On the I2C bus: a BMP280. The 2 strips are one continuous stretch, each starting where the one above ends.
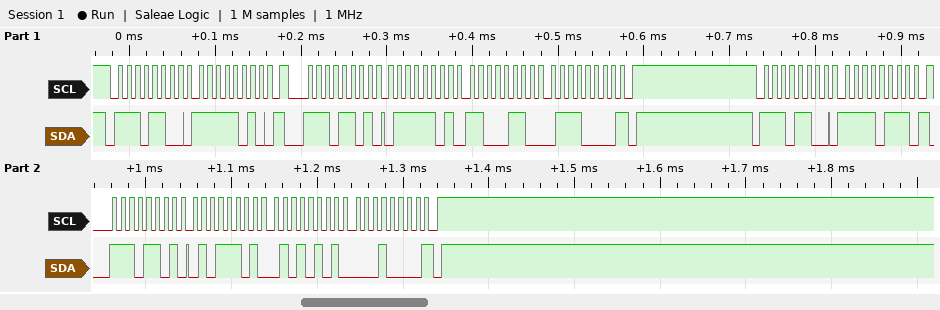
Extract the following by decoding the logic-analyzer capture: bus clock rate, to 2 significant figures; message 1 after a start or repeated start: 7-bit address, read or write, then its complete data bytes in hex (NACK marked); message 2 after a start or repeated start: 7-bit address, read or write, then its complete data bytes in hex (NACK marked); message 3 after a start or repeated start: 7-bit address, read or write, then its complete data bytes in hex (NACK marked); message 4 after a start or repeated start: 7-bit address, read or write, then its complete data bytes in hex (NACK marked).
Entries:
100 kHz
0x76 write: FA
0x76 read: 7D C6 70 NACK
0x76 write: F7
0x76 read: 5D 55 10 NACK
